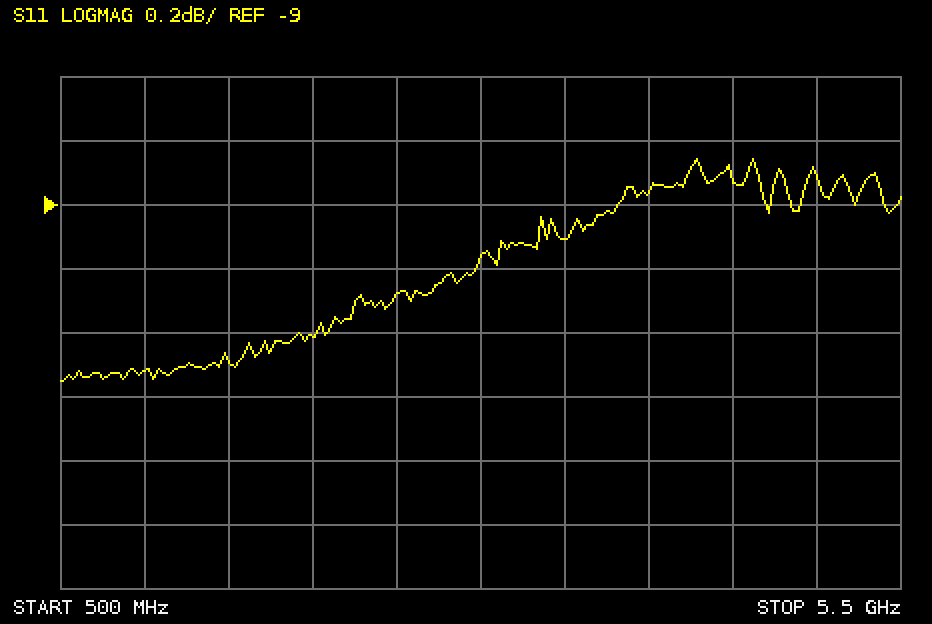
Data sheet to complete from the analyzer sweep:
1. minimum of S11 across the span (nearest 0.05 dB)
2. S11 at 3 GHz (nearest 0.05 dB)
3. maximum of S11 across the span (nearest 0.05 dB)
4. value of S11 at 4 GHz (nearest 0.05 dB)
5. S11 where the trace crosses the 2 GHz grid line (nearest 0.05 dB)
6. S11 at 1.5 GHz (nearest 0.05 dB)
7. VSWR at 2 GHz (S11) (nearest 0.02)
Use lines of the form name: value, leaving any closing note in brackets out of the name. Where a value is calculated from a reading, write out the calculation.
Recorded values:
minimum of S11 across the span: -9.55 dB
S11 at 3 GHz: -9.15 dB
maximum of S11 across the span: -8.85 dB
value of S11 at 4 GHz: -8.95 dB
S11 where the trace crosses the 2 GHz grid line: -9.40 dB
S11 at 1.5 GHz: -9.50 dB
VSWR at 2 GHz (S11): |Γ| = 10^(-9.4/20) = 0.3388; VSWR = (1 + 0.3388)/(1 − 0.3388) ≈ 2.03, so 2.02 to the nearest 0.02
